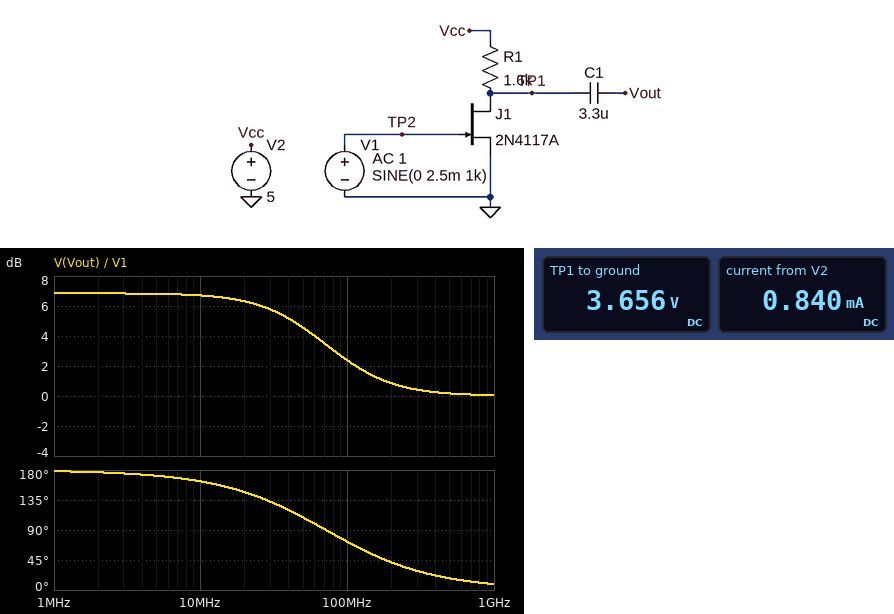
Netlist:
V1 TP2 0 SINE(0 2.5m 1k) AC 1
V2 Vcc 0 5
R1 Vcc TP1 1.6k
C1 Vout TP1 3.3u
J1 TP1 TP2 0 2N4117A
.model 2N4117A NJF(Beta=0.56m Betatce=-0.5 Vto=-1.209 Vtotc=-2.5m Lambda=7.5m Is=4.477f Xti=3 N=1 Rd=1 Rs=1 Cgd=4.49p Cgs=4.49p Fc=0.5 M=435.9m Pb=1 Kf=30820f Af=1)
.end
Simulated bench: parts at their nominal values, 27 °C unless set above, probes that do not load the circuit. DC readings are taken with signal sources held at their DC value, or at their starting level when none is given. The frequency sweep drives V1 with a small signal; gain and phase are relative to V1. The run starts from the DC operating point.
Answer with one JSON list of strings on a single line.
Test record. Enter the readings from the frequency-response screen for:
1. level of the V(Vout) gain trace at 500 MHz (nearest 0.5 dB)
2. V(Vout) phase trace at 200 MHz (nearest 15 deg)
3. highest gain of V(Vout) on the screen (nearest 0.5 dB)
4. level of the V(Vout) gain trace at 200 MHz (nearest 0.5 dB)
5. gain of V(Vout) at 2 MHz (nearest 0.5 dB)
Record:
["0 dB", "45 deg", "7.0 dB", "1.0 dB", "7.0 dB"]
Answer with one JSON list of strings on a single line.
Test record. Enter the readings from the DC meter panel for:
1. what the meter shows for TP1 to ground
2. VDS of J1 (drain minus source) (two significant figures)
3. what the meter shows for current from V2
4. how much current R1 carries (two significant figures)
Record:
["3.656 V", "3.7 V", "0.840 mA", "840 µA"]
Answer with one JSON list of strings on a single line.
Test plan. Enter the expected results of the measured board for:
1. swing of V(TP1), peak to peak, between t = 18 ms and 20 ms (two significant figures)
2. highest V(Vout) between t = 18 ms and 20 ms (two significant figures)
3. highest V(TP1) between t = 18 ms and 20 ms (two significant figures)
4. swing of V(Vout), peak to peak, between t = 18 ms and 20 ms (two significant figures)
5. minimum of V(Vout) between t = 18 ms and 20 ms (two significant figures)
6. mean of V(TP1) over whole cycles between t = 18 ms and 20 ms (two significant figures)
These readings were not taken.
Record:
["11 mV", "5.5 mV", "3.7 V", "11 mV", "-5.5 mV", "3.7 V"]
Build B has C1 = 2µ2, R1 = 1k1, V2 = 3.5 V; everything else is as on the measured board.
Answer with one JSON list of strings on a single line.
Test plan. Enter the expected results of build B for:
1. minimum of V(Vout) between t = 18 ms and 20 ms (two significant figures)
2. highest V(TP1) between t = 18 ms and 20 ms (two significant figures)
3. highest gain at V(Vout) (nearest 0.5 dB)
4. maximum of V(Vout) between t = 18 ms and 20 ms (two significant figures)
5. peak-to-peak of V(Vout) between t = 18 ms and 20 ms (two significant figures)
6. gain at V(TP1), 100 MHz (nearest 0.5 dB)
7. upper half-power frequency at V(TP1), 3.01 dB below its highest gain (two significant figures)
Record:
["-3.8 mV", "2.6 V", "3.5 dB", "3.8 mV", "7.5 mV", "1.5 dB", "180 MHz"]
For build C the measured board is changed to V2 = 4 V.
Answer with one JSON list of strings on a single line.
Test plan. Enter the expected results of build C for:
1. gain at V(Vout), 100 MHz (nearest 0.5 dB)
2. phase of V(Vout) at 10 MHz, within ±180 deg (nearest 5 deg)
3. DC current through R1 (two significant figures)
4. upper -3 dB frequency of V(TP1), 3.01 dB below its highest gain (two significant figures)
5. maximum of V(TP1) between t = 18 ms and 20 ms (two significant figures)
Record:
["2.0 dB", "160 deg", "830 µA", "56 MHz", "2.7 V"]
